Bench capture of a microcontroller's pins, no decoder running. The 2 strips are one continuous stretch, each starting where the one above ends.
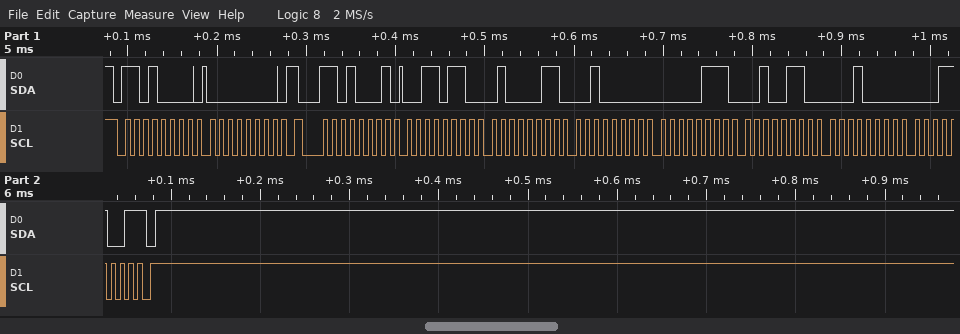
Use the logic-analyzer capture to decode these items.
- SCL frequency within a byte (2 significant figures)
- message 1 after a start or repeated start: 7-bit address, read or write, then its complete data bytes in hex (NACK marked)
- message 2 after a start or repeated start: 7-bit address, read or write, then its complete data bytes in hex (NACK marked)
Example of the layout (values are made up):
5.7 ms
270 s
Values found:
100 kHz
0x68 write: 00
0x68 read: 36 43 20 07 26 10 19 NACK
